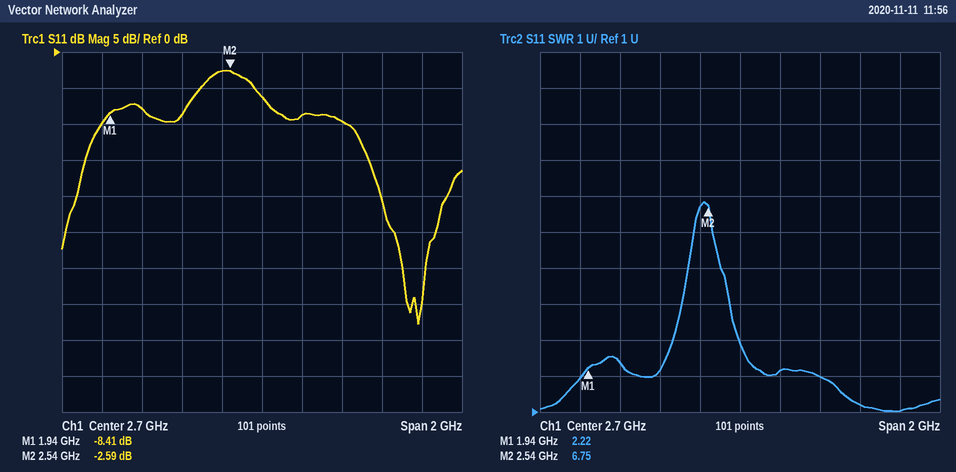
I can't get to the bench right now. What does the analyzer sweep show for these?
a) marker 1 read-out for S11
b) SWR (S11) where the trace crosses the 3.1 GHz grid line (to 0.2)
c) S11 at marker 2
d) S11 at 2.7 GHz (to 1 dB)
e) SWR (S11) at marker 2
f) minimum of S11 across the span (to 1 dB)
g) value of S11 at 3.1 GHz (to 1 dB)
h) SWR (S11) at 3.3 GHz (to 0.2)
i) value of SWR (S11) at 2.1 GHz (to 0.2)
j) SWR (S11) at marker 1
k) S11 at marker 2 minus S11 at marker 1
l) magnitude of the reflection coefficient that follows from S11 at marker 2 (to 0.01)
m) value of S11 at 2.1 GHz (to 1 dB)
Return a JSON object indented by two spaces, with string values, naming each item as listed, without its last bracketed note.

{
  "marker 1 read-out for S11": "-8.41 dB",
  "SWR (S11) where the trace crosses the 3.1 GHz grid line": "2.0",
  "S11 at marker 2": "-2.59 dB",
  "S11 at 2.7 GHz": "-6 dB",
  "SWR (S11) at marker 2": "6.75",
  "minimum of S11 across the span": "-38 dB",
  "value of S11 at 3.1 GHz": "-10 dB",
  "SWR (S11) at 3.3 GHz": "1.2",
  "value of SWR (S11) at 2.1 GHz": "2.4",
  "SWR (S11) at marker 1": "2.22",
  "S11 at marker 2 minus S11 at marker 1": "5.82 dB",
  "magnitude of the reflection coefficient that follows from S11 at marker 2": "0.74",
  "value of S11 at 2.1 GHz": "-8 dB"
}
